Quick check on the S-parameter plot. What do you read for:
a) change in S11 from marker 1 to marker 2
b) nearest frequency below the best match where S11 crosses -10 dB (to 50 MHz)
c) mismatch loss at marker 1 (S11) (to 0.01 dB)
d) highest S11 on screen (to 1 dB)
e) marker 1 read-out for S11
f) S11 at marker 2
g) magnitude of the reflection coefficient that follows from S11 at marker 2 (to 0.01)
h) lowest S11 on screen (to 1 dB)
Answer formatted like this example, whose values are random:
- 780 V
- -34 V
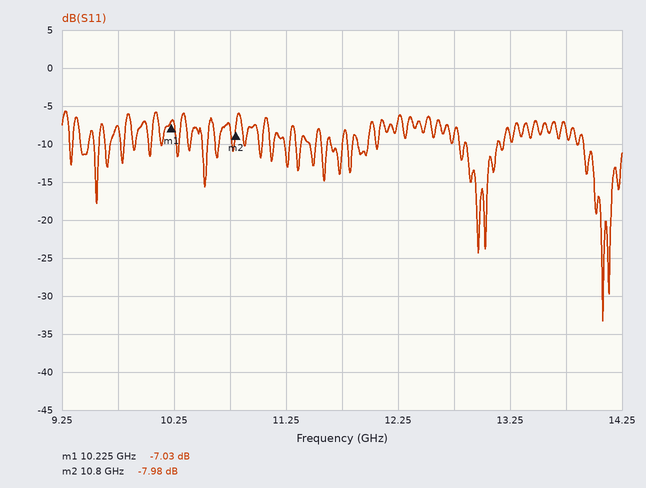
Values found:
- -0.95 dB
- 13.90 GHz
- 0.96 dB
- -6 dB
- -7.03 dB
- -7.98 dB
- 0.40
- -33 dB
